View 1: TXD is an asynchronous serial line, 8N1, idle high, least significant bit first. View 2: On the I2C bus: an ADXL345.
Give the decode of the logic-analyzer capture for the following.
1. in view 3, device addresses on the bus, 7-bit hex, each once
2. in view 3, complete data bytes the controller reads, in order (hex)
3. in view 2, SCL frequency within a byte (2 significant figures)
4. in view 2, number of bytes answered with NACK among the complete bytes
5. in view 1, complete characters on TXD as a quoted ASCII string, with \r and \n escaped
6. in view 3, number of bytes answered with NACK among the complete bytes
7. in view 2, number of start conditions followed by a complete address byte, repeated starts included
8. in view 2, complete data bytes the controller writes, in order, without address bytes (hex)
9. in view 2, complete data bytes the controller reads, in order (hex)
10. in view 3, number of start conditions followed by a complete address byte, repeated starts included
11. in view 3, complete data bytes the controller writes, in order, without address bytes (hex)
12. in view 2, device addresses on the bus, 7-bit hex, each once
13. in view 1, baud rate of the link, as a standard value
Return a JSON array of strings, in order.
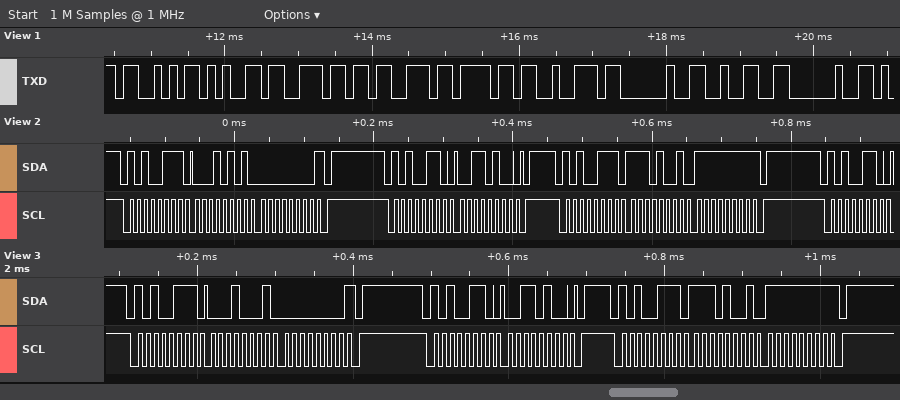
["0x53", "11 00 E9 FF", "100 kHz", "2", "\"Sensor 2 \"", "2", "4", "34", "15 00 E9 FF", "3", "34", "0x53", "9600 baud"]
